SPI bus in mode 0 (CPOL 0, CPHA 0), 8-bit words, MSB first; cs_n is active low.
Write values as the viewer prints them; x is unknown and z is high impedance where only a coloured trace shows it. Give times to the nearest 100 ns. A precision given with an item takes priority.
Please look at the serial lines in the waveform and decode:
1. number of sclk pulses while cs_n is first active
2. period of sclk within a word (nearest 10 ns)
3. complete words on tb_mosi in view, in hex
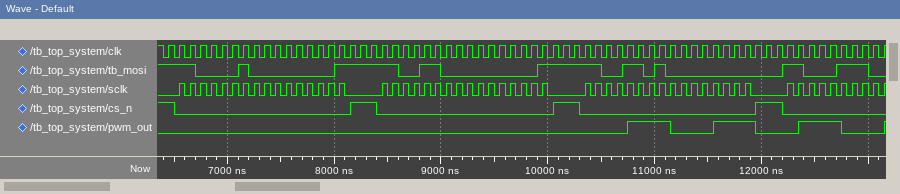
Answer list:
16
100 ns
C2, 01, CC, 01, CD, 00, C7
